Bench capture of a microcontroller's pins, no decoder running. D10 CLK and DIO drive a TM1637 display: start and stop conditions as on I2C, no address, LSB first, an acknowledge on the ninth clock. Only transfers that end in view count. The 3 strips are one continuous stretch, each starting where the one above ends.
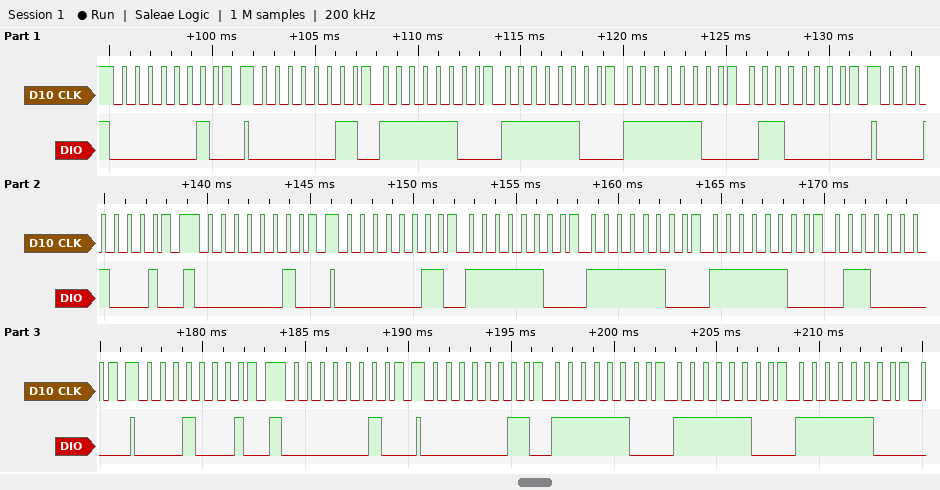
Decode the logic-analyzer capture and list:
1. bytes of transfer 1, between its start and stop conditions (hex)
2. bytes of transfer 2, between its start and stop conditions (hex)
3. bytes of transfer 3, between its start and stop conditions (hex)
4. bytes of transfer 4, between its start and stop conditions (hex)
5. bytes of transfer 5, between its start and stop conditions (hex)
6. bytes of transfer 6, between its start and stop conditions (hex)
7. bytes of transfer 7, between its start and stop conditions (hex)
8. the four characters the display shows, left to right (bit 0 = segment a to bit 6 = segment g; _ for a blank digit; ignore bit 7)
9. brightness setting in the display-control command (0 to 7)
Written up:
40
C0 3F 3F 3F 06
88
40
C0 3F 3F 3F 06
88
40
0001
0
